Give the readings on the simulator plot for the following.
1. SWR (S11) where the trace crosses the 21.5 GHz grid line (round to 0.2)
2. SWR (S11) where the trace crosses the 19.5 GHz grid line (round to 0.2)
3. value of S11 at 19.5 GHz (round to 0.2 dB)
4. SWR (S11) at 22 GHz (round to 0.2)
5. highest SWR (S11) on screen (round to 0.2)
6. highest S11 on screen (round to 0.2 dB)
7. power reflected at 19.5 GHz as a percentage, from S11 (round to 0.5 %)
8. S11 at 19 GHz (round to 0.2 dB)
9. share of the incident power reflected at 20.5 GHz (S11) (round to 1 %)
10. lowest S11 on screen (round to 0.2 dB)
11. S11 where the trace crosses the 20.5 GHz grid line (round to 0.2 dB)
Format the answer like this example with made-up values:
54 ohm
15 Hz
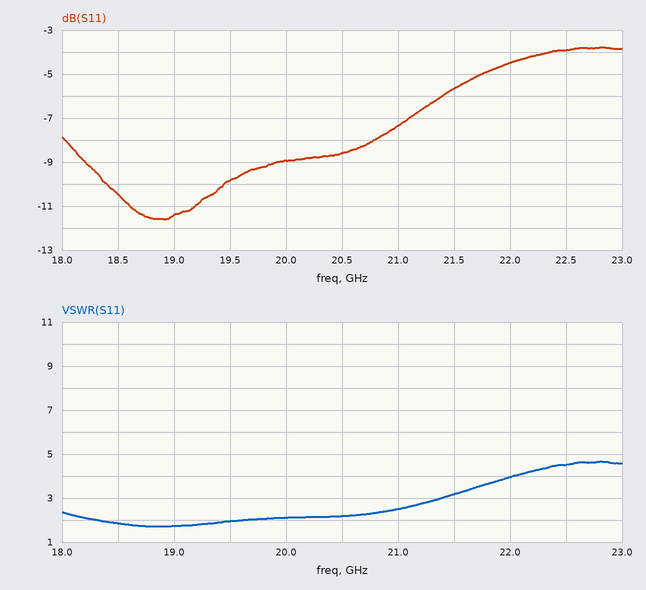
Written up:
3.2
2.0
-9.8 dB
4.0
4.6
-3.8 dB
10.5 %
-11.4 dB
14 %
-11.6 dB
-8.6 dB
